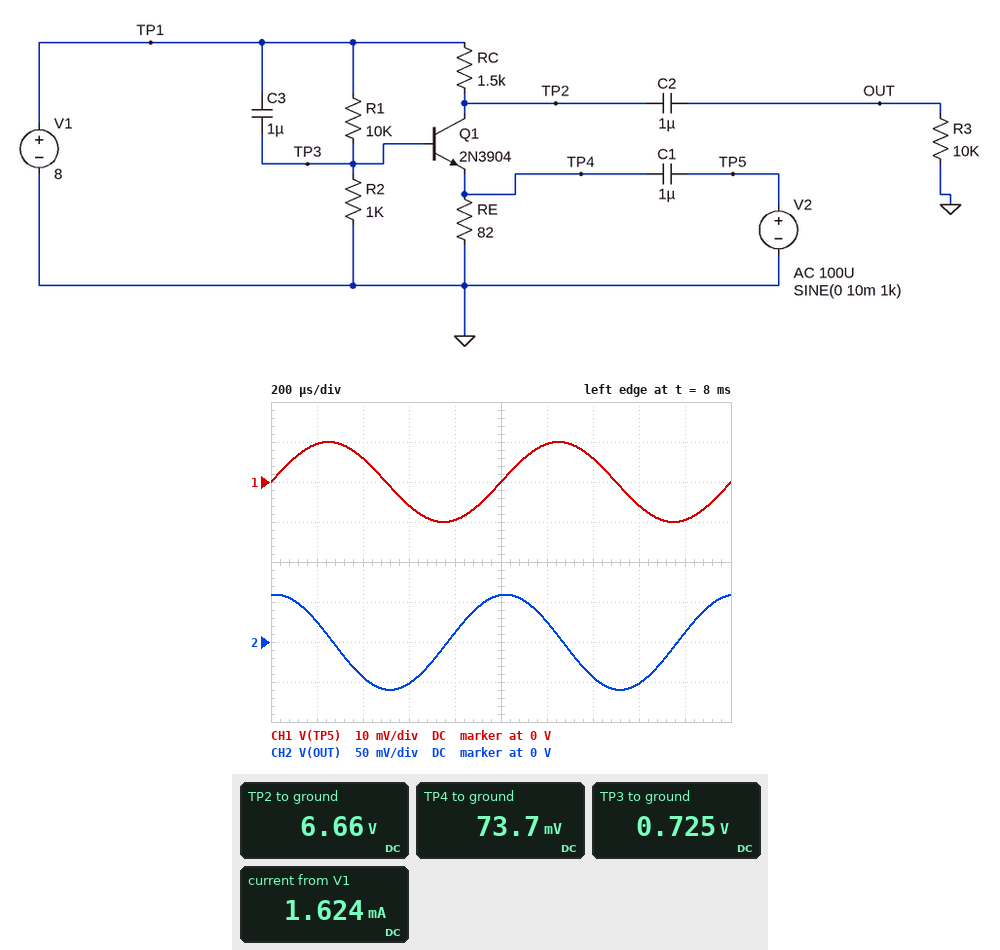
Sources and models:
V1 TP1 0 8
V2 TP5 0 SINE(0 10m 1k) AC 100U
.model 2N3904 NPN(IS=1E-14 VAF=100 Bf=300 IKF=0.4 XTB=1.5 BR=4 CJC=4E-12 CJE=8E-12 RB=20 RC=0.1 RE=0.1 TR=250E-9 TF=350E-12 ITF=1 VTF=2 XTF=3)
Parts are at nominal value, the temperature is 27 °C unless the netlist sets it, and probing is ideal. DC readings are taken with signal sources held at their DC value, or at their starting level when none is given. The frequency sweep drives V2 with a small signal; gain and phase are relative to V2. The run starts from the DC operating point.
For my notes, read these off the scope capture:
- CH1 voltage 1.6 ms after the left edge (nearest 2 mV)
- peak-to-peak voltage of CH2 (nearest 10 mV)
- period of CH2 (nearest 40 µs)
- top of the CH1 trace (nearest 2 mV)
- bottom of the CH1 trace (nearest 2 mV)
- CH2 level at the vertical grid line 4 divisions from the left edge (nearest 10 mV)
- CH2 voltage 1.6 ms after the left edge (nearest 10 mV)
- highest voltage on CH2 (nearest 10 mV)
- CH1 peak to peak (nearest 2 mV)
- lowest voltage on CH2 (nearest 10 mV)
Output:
-6 mV
120 mV
1.00 ms
10 mV
-10 mV
10 mV
-50 mV
60 mV
20 mV
-60 mV
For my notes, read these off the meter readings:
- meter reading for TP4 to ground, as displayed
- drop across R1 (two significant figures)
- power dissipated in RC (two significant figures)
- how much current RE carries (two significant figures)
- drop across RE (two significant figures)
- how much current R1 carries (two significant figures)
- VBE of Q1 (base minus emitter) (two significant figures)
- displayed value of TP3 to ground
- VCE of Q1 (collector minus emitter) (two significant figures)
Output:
73.7 mV
7.3 V
1.2 mW
900 µA
74 mV
730 µA
650 mV
0.725 V
6.6 V
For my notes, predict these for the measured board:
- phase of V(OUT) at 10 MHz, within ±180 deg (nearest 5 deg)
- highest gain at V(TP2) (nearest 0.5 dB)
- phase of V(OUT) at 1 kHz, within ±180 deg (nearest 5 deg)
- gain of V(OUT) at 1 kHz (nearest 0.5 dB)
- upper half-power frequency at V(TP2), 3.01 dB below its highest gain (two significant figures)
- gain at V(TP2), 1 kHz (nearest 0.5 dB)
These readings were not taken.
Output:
-15 deg
33.0 dB
85 deg
15.5 dB
35 MHz
15.5 dB
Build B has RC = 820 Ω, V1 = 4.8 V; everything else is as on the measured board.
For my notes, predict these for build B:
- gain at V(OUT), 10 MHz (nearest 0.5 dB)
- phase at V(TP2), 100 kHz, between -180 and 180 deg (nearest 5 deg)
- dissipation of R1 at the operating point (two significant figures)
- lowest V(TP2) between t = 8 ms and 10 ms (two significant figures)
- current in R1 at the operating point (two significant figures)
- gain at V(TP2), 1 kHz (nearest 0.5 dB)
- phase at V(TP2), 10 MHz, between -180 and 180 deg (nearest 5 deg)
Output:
-46.0 dB
0 deg
1.9 mW
4.8 V
440 µA
-50.5 dB
-5 deg
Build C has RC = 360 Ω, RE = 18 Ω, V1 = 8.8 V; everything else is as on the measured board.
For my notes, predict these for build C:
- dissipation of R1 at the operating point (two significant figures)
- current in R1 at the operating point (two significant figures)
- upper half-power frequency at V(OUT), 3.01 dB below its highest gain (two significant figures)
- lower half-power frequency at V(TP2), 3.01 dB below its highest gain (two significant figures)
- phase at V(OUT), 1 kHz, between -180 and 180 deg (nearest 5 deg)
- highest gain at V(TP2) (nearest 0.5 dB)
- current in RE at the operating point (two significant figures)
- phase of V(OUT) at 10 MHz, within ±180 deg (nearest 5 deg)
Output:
6.4 mW
800 µA
36 MHz
38 kHz
90 deg
36.0 dB
5.0 mA
-15 deg
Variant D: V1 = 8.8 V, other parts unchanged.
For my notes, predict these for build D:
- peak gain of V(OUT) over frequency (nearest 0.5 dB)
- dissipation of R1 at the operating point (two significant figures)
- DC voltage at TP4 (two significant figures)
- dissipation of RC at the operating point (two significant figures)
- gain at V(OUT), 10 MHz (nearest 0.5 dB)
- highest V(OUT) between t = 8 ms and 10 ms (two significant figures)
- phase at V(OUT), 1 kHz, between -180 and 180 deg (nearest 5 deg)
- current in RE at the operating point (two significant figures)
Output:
37.5 dB
6.4 mW
130 mV
3.7 mW
37.0 dB
67 mV
85 deg
1.6 mA
